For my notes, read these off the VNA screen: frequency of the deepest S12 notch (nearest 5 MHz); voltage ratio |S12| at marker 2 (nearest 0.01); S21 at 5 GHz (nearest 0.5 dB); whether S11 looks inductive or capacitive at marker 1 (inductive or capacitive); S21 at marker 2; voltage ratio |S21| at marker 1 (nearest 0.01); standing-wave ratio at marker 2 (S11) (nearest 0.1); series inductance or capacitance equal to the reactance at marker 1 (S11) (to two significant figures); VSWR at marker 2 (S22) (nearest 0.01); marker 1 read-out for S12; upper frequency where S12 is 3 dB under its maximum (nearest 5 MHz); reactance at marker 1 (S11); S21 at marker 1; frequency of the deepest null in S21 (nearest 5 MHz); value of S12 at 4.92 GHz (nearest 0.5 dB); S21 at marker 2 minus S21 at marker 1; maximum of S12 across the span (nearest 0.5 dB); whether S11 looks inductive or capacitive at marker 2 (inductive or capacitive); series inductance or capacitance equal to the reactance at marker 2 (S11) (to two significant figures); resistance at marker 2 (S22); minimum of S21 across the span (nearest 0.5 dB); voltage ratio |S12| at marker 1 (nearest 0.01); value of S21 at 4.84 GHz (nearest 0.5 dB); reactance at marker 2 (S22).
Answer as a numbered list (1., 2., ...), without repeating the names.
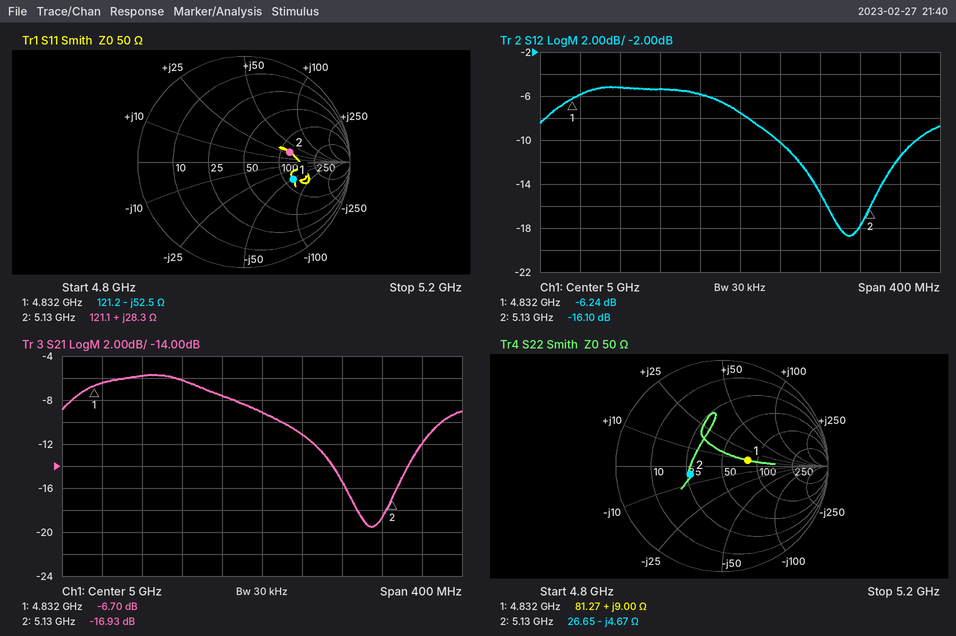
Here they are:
1. 5.110 GHz
2. 0.16
3. -9.0 dB
4. capacitive
5. -16.93 dB
6. 0.46
7. 2.6
8. 630 fF
9. 1.90
10. -6.24 dB
11. 5.010 GHz
12. -52.5 Ω
13. -6.70 dB
14. 5.110 GHz
15. -5.5 dB
16. -10.23 dB
17. -5.0 dB
18. inductive
19. 880 pH
20. 26.65 Ω
21. -19.5 dB
22. 0.49
23. -6.5 dB
24. -4.67 Ω
